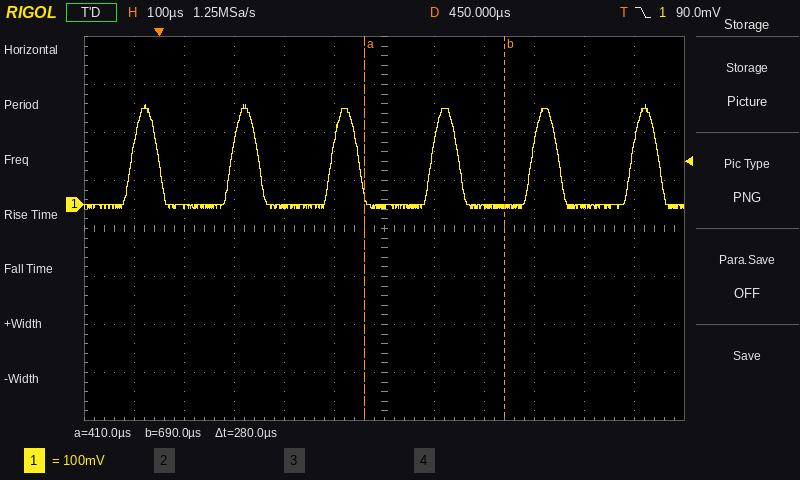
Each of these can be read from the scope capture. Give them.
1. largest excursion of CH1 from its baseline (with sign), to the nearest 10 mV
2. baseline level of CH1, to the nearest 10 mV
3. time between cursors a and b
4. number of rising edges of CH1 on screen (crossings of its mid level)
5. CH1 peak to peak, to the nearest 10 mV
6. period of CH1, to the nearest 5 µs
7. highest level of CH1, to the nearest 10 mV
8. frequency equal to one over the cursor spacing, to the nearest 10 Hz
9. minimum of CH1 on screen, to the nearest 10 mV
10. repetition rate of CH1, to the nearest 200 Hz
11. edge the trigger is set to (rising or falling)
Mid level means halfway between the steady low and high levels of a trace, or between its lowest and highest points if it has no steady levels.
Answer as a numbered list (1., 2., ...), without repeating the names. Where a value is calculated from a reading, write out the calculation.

1. 210 mV − (0 mV) = +210 mV
2. 0 mV
3. 280 µs
4. 6
5. 210 mV − (-10 mV) = 220 mV
6. 200 µs
7. 210 mV
8. 1 / 280 µs ≈ 3.57 kHz
9. -10 mV
10. 1 / 200 µs ≈ 5.0 kHz
11. falling
